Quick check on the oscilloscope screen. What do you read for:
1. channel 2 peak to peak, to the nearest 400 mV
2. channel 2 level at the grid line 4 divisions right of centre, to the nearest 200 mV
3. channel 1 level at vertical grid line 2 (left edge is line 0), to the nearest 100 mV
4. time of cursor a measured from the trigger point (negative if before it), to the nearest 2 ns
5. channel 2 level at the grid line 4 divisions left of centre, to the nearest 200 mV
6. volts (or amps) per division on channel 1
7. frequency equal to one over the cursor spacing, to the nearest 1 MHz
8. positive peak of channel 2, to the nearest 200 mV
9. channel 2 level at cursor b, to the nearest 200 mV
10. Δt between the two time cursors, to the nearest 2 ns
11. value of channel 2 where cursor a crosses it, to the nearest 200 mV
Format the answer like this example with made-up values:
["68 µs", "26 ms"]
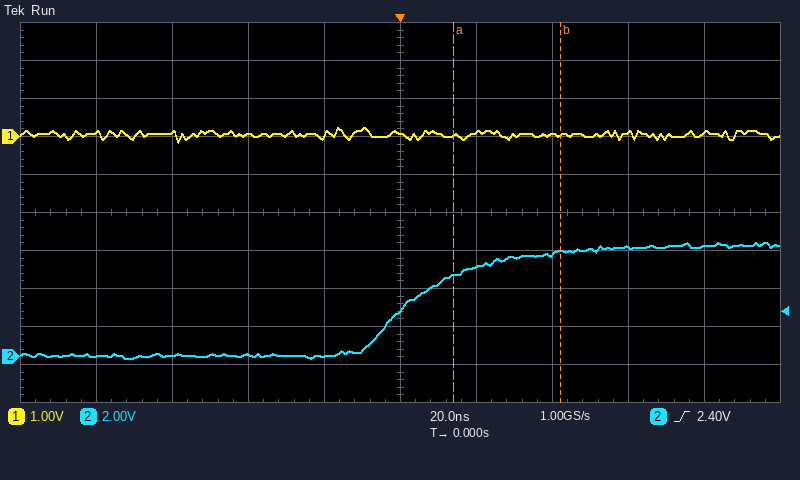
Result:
["6.0 V", "5.8 V", "100 mV", "+14 ns", "0.0 V", "1 V", "36 MHz", "6.0 V", "5.6 V", "28 ns", "4.2 V"]
